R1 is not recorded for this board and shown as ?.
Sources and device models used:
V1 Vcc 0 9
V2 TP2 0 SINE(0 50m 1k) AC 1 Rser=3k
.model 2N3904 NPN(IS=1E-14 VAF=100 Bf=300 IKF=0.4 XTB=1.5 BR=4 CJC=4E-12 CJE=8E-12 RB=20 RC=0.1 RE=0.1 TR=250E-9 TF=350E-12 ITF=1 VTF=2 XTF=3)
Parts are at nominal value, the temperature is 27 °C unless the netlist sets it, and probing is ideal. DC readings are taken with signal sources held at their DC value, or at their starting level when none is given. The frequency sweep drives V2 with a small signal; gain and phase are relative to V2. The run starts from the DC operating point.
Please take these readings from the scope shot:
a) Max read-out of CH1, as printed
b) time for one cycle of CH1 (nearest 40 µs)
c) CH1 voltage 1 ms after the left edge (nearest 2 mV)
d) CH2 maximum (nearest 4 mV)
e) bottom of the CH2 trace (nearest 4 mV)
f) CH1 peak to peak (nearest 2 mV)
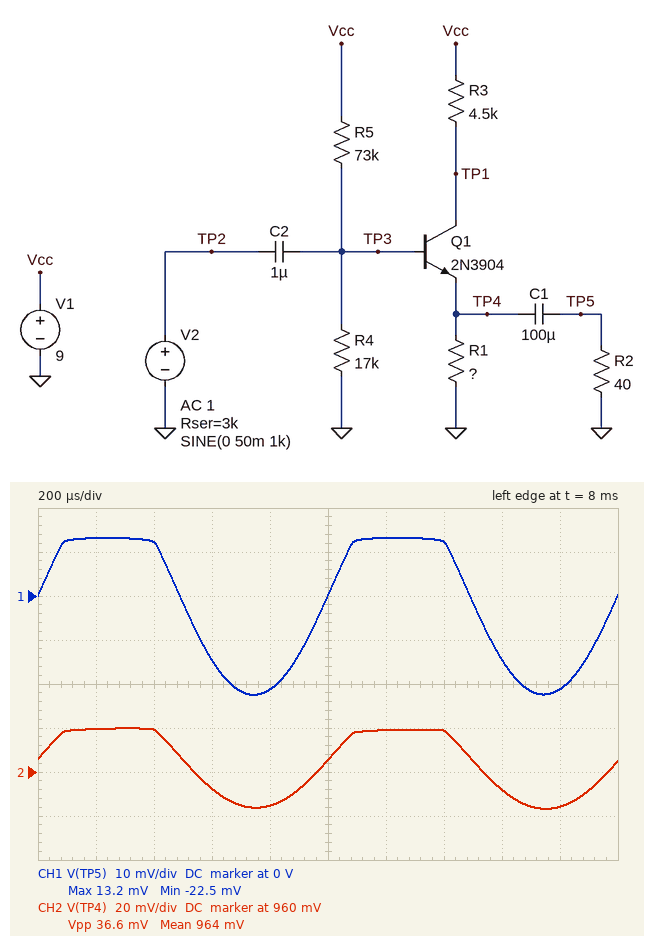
13.2 mV
1.00 ms
0 V
980 mV
944 mV
36 mV
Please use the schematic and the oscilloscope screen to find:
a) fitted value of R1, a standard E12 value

680 Ω
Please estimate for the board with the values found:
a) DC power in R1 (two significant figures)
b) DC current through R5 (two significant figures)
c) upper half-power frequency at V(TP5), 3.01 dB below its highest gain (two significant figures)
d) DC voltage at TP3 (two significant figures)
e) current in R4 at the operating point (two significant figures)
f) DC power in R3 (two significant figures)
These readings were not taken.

1.4 mW
100 µA
290 kHz
1.6 V
96 µA
9.1 mW
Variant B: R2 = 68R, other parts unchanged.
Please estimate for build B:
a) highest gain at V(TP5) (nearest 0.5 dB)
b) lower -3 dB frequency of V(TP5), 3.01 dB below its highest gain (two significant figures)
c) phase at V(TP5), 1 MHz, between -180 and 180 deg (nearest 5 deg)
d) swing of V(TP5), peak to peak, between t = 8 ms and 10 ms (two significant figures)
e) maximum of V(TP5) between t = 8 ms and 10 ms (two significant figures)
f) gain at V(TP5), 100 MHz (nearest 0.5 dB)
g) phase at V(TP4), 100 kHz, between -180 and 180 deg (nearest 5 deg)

-5.0 dB
25 Hz
-65 deg
49 mV
21 mV
-34.5 dB
-15 deg
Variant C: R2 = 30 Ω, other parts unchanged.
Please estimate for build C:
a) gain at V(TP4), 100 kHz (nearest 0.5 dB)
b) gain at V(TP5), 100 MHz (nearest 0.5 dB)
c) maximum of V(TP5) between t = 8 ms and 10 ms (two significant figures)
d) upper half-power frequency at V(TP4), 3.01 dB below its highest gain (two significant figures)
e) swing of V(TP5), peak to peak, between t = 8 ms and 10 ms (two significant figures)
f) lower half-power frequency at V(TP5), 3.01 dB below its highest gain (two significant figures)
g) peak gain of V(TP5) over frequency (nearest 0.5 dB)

-8.5 dB
-41.0 dB
10 mV
120 kHz
29 mV
38 Hz
-7.5 dB
